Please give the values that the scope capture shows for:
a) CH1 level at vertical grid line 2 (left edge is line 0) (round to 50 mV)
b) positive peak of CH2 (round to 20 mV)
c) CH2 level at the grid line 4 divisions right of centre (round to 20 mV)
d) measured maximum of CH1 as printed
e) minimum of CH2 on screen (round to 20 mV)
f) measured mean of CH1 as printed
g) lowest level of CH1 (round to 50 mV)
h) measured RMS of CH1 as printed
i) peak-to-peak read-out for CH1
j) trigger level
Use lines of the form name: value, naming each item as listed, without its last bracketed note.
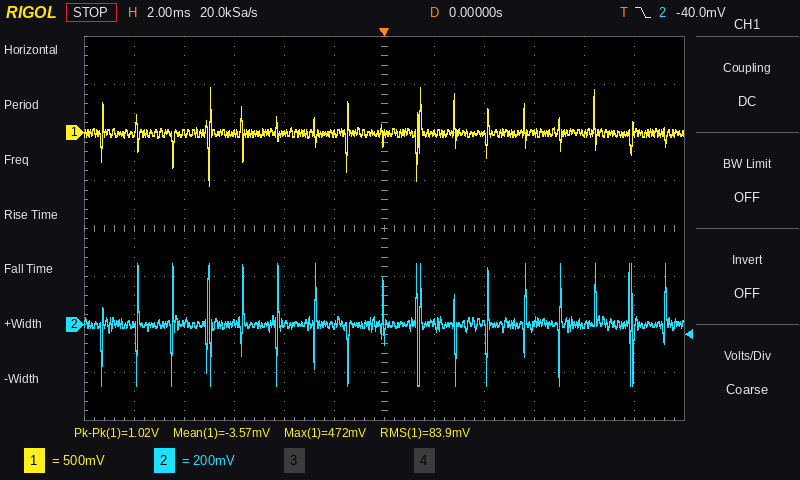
CH1 level at vertical grid line 2 (left edge is line 0): 0 mV
positive peak of CH2: 260 mV
CH2 level at the grid line 4 divisions right of centre: 0 mV
measured maximum of CH1 as printed: 472 mV
minimum of CH2 on screen: -260 mV
measured mean of CH1 as printed: -3.57 mV
lowest level of CH1: -550 mV
measured RMS of CH1 as printed: 83.9 mV
peak-to-peak read-out for CH1: 1.02 V
trigger level: -40.0 mV
